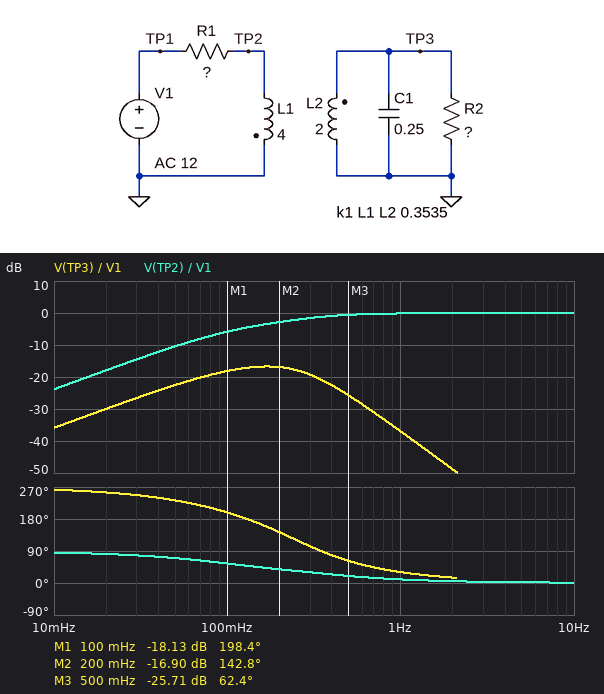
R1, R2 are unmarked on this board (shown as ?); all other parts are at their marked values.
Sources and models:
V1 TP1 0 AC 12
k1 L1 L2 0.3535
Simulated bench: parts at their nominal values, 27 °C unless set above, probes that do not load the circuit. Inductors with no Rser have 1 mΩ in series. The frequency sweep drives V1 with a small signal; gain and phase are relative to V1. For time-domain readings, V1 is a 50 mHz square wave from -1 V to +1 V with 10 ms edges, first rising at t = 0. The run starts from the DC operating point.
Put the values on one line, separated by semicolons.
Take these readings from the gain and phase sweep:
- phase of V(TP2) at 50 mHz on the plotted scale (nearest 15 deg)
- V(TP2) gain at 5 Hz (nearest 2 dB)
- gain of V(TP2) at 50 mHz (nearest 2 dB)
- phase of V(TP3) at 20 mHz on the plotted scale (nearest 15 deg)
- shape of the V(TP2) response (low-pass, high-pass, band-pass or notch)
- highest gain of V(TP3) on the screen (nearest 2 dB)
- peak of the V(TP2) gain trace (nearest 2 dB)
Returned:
75 deg; 0 dB; -10 dB; 255 deg; high-pass; -16 dB; 0 dB
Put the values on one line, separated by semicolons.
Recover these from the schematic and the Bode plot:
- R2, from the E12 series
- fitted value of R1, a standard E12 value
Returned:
1.8 Ω; 3.9 Ω
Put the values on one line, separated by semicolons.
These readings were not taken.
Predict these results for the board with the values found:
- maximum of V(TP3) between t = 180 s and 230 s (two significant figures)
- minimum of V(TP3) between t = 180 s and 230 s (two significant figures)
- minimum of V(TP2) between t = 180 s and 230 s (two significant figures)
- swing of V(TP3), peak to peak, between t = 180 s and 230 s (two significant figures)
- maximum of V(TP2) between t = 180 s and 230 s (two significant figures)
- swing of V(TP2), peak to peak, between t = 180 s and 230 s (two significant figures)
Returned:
200 mV; -200 mV; -2.0 V; 400 mV; 2.0 V; 4.0 V
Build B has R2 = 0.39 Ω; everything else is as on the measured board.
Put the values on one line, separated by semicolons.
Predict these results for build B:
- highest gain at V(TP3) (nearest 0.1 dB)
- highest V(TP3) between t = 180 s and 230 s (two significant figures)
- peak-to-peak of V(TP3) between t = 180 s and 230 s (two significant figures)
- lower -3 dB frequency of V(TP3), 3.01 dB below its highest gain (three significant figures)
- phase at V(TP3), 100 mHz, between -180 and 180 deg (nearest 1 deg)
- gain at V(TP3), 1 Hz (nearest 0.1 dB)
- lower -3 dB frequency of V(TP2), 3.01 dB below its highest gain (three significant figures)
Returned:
-27.5 dB; 59 mV; 120 mV; 23.7 mHz; 165 deg; -42.4 dB; 181 mHz
